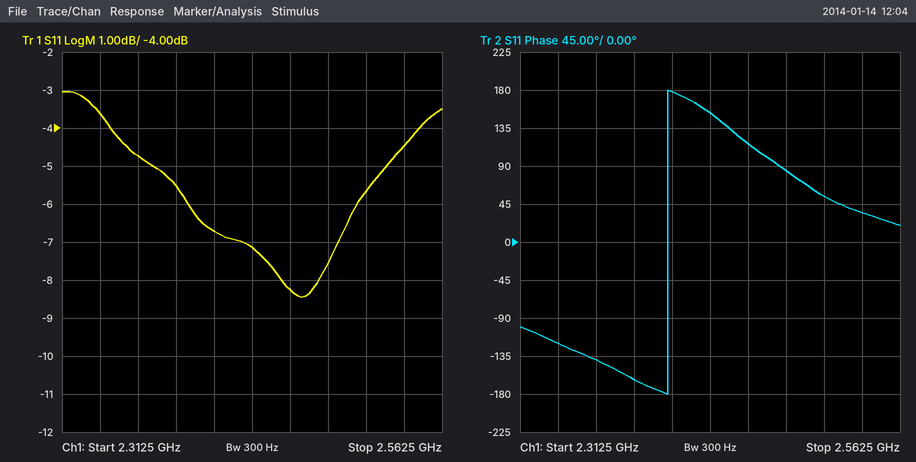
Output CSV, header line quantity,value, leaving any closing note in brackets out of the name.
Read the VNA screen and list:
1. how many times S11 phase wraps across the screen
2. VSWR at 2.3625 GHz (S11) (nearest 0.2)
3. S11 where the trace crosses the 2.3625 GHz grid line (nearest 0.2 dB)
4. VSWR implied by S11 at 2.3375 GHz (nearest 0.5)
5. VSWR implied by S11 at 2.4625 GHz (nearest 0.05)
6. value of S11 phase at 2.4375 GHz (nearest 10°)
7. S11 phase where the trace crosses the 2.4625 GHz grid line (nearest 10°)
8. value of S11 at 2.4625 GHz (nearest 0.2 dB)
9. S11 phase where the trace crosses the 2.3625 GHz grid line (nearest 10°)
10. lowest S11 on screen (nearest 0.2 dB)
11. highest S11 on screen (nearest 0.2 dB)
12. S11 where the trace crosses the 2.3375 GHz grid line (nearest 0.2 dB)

quantity,value
how many times S11 phase wraps across the screen,1
VSWR at 2.3625 GHz (S11),3.8
S11 where the trace crosses the 2.3625 GHz grid line,-4.8 dB
VSWR implied by S11 at 2.3375 GHz,5.0
VSWR implied by S11 at 2.4625 GHz,2.25
value of S11 phase at 2.4375 GHz,150°
S11 phase where the trace crosses the 2.4625 GHz grid line,120°
value of S11 at 2.4625 GHz,-8.2 dB
S11 phase where the trace crosses the 2.3625 GHz grid line,-140°
lowest S11 on screen,-8.4 dB
highest S11 on screen,-3.0 dB
S11 where the trace crosses the 2.3375 GHz grid line,-3.6 dB
